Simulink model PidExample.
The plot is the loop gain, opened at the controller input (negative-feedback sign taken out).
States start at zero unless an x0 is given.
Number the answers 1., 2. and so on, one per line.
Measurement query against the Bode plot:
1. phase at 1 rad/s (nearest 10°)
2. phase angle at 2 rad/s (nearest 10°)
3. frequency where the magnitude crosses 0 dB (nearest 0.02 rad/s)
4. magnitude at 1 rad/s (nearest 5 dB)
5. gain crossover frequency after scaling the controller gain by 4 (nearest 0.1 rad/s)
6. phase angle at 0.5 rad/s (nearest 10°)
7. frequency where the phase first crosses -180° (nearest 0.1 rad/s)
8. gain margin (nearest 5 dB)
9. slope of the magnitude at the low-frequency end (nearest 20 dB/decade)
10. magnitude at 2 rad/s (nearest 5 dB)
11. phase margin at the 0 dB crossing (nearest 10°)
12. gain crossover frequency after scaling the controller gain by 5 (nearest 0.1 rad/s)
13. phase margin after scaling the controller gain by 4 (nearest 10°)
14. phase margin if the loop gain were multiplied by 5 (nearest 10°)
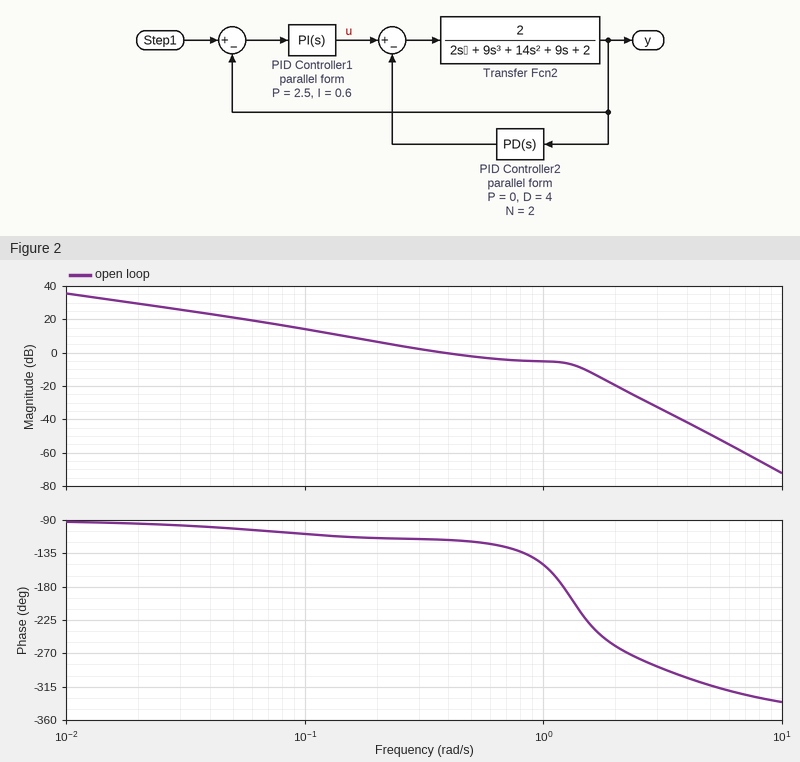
1. -150°
2. -260°
3. 0.38 rad/s
4. -5 dB
5. 1.6 rad/s
6. -120°
7. 1.2 rad/s
8. 5 dB
9. -20 dB/decade
10. -20 dB
11. 60°
12. 1.7 rad/s
13. -50°
14. -60°
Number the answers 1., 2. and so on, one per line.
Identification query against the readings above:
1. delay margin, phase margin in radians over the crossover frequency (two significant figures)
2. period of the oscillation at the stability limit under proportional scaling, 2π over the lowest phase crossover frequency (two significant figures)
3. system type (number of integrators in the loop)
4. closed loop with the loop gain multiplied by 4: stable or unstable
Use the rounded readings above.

1. 2.8 s
2. 5.2 s
3. 1
4. unstable
